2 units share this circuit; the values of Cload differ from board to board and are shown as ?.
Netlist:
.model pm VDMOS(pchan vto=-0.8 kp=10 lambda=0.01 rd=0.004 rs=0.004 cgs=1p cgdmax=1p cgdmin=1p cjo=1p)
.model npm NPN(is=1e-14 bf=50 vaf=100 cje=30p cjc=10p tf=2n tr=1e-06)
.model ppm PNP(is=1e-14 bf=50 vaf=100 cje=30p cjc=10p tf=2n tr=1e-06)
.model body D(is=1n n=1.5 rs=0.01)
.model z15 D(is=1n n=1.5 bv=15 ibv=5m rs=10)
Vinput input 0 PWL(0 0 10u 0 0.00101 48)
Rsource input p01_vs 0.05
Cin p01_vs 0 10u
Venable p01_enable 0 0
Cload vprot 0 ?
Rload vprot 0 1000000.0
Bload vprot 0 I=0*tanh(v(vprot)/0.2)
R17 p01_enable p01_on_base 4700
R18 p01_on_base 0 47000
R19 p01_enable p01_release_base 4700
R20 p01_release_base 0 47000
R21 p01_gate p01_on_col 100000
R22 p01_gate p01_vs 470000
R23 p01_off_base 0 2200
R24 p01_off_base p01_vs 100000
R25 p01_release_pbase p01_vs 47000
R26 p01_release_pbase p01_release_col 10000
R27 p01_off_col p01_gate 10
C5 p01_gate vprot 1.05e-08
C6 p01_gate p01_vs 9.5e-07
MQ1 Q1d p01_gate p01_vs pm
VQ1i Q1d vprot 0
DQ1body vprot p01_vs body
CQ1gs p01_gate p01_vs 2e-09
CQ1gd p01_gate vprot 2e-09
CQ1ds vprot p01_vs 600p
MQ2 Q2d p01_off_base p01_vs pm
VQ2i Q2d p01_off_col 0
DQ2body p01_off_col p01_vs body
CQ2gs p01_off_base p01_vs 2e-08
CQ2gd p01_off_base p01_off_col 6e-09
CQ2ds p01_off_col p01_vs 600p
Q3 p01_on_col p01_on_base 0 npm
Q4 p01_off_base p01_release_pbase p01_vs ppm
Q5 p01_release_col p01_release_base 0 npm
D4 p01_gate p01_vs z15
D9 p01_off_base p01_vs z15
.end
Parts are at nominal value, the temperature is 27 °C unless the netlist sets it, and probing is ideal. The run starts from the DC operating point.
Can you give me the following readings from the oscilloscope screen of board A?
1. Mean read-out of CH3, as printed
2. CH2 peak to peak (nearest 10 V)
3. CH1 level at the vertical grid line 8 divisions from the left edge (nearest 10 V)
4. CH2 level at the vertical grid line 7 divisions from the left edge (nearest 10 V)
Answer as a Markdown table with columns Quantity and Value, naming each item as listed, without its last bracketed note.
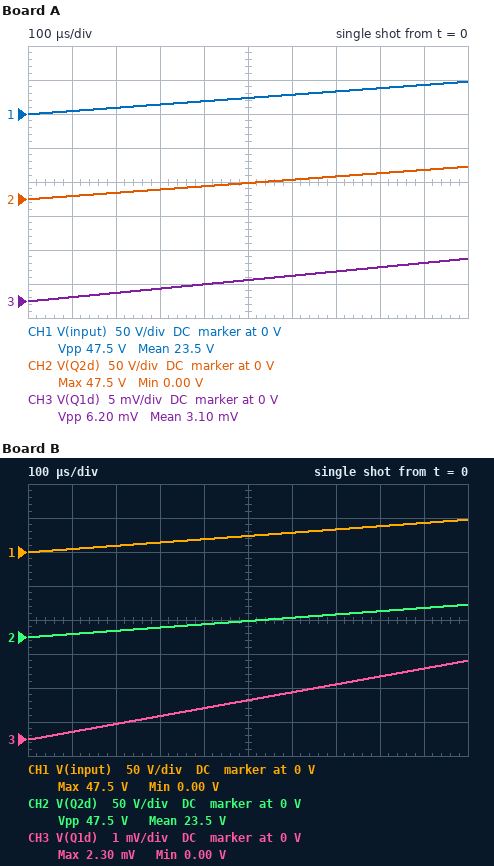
| Quantity | Value |
|---|---|
| Mean read-out of CH3, as printed | 3.10 mV |
| CH2 peak to peak | 50 V |
| CH1 level at the vertical grid line 8 divisions from the left edge | 40 V |
| CH2 level at the vertical grid line 7 divisions from the left edge | 30 V |
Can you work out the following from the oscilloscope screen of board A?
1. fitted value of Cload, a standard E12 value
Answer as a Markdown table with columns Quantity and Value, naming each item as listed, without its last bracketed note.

| Quantity | Value |
|---|---|
| fitted value of Cload, a standard E12 value | 100 µF |
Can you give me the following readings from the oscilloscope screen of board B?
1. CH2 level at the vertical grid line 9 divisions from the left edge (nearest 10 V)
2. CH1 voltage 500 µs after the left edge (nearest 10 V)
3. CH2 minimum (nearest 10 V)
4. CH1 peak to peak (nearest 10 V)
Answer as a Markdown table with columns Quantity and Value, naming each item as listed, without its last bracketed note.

| Quantity | Value |
|---|---|
| CH2 level at the vertical grid line 9 divisions from the left edge | 40 V |
| CH1 voltage 500 µs after the left edge | 20 V |
| CH2 minimum | 0 V |
| CH1 peak to peak | 50 V |
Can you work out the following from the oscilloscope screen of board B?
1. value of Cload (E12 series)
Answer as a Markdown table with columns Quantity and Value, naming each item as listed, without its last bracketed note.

| Quantity | Value |
|---|---|
| value of Cload | 270 µF |
